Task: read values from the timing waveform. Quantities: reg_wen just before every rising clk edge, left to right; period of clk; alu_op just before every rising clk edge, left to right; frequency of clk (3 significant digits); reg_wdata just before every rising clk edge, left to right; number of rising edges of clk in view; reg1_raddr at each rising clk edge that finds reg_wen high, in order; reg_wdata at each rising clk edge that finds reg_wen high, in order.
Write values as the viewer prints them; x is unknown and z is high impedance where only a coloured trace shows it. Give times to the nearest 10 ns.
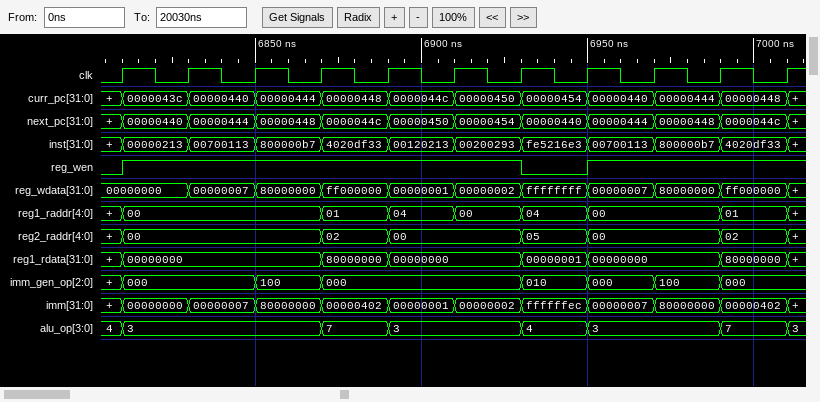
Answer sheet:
0 1 1 1 1 1 1 0 1 1 1
20 ns
4, 3, 3, 3, 7, 3, 3, 4, 3, 3, 7
50.0 MHz
00000000, 00000000, 00000007, 80000000, ff000000, 00000001, 00000002, ffffffff, 00000007, 80000000, ff000000
11
00, 00, 00, 01, 04, 00, 00, 00, 01
00000000, 00000007, 80000000, ff000000, 00000001, 00000002, 00000007, 80000000, ff000000
